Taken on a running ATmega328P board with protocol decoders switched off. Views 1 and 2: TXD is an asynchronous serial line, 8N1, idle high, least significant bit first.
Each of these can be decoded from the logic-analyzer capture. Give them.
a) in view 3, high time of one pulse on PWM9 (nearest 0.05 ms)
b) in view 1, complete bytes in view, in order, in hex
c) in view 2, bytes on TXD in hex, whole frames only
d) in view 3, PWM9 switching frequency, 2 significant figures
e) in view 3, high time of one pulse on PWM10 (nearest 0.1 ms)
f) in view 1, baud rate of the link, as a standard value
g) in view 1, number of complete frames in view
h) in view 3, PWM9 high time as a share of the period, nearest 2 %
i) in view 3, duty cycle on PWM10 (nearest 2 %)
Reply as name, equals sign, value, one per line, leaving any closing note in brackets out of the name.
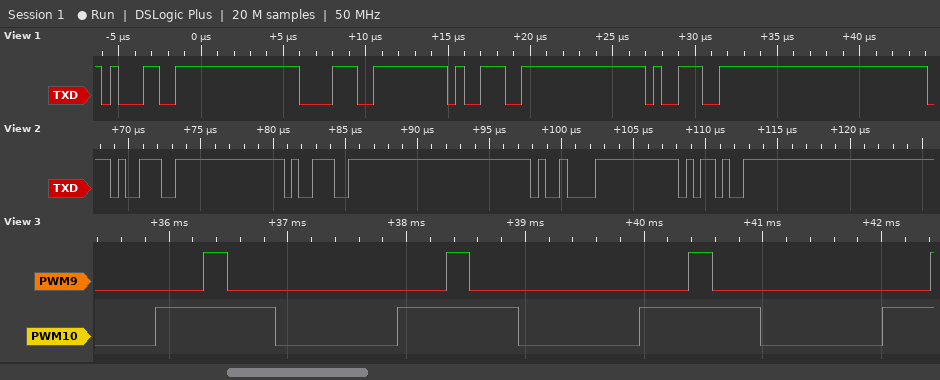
in view 3, high time of one pulse on PWM9 = 0.20 ms
in view 1, complete bytes in view, in order, in hex = 0x31 0x38 0x39 0x39
in view 2, bytes on TXD in hex, whole frames only = 39 39 09 2D
in view 3, PWM9 switching frequency, 2 significant figures = 490 Hz
in view 3, high time of one pulse on PWM10 = 1.0 ms
in view 1, baud rate of the link, as a standard value = 2000000 baud
in view 1, number of complete frames in view = 4
in view 3, PWM9 high time as a share of the period, nearest 2 % = 10 %
in view 3, duty cycle on PWM10 = 50 %
